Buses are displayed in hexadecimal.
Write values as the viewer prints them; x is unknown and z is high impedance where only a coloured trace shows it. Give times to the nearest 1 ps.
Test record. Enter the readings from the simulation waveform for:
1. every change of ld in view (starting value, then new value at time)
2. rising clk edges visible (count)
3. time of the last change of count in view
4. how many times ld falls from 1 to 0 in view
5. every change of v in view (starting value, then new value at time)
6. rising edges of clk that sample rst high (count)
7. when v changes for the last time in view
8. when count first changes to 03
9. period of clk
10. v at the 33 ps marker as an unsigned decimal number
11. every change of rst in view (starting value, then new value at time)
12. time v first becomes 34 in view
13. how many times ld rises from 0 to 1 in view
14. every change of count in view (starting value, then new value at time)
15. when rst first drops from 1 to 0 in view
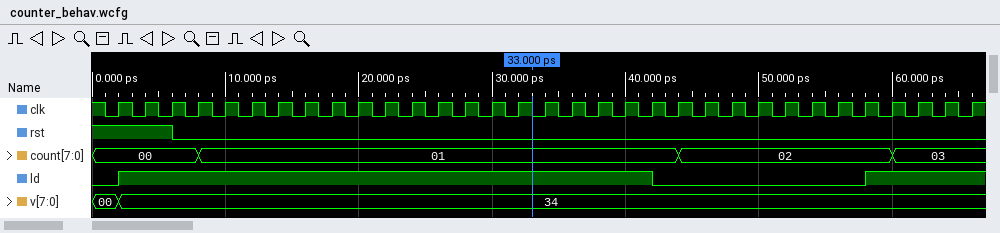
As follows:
0, 1 at 2 ps, 0 at 42 ps, 1 at 58 ps
33
60 ps
1
00, 34 at 2 ps
3
2 ps
60 ps
2 ps
52
1, 0 at 6 ps
2 ps
2
00, 01 at 8 ps, 02 at 44 ps, 03 at 60 ps
6 ps
